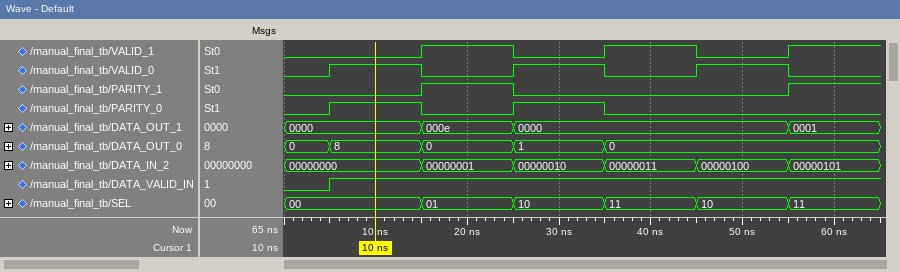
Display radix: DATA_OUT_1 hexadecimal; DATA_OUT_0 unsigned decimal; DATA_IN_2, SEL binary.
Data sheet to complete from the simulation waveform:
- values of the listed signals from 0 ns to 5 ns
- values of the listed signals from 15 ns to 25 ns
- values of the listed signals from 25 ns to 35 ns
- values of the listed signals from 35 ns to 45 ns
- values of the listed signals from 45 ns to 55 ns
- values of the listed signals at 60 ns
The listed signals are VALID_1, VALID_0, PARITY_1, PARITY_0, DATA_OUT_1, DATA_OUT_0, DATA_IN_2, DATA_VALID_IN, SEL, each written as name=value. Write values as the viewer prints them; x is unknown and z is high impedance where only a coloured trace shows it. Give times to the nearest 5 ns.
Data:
VALID_1=0, VALID_0=0, PARITY_1=0, PARITY_0=0, DATA_OUT_1=0000, DATA_OUT_0=0, DATA_IN_2=00000000, DATA_VALID_IN=0, SEL=00
VALID_1=1, VALID_0=0, PARITY_1=1, PARITY_0=0, DATA_OUT_1=000e, DATA_OUT_0=0, DATA_IN_2=00000001, DATA_VALID_IN=1, SEL=01
VALID_1=0, VALID_0=1, PARITY_1=0, PARITY_0=1, DATA_OUT_1=0000, DATA_OUT_0=1, DATA_IN_2=00000010, DATA_VALID_IN=1, SEL=10
VALID_1=1, VALID_0=0, PARITY_1=0, PARITY_0=0, DATA_OUT_1=0000, DATA_OUT_0=0, DATA_IN_2=00000011, DATA_VALID_IN=1, SEL=11
VALID_1=0, VALID_0=1, PARITY_1=0, PARITY_0=0, DATA_OUT_1=0000, DATA_OUT_0=0, DATA_IN_2=00000100, DATA_VALID_IN=1, SEL=10
VALID_1=1, VALID_0=0, PARITY_1=1, PARITY_0=0, DATA_OUT_1=0001, DATA_OUT_0=0, DATA_IN_2=00000101, DATA_VALID_IN=1, SEL=11
